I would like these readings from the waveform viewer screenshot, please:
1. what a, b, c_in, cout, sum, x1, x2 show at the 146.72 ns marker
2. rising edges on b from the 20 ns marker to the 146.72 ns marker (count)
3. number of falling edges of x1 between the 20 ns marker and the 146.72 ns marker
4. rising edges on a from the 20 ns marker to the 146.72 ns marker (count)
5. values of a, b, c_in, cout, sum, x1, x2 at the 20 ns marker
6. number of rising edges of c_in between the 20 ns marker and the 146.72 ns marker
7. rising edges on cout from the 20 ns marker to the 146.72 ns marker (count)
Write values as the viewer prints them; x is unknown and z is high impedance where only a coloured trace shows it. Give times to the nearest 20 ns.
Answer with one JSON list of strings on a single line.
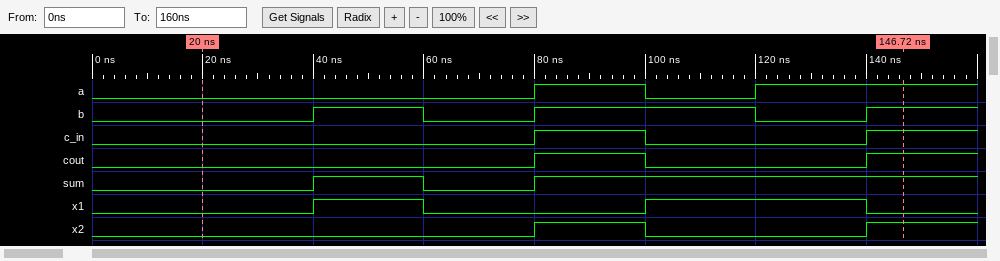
["a=1, b=1, c_in=1, cout=1, sum=1, x1=0, x2=1", "3", "2", "2", "a=0, b=0, c_in=0, cout=0, sum=0, x1=0, x2=0", "2", "2"]
